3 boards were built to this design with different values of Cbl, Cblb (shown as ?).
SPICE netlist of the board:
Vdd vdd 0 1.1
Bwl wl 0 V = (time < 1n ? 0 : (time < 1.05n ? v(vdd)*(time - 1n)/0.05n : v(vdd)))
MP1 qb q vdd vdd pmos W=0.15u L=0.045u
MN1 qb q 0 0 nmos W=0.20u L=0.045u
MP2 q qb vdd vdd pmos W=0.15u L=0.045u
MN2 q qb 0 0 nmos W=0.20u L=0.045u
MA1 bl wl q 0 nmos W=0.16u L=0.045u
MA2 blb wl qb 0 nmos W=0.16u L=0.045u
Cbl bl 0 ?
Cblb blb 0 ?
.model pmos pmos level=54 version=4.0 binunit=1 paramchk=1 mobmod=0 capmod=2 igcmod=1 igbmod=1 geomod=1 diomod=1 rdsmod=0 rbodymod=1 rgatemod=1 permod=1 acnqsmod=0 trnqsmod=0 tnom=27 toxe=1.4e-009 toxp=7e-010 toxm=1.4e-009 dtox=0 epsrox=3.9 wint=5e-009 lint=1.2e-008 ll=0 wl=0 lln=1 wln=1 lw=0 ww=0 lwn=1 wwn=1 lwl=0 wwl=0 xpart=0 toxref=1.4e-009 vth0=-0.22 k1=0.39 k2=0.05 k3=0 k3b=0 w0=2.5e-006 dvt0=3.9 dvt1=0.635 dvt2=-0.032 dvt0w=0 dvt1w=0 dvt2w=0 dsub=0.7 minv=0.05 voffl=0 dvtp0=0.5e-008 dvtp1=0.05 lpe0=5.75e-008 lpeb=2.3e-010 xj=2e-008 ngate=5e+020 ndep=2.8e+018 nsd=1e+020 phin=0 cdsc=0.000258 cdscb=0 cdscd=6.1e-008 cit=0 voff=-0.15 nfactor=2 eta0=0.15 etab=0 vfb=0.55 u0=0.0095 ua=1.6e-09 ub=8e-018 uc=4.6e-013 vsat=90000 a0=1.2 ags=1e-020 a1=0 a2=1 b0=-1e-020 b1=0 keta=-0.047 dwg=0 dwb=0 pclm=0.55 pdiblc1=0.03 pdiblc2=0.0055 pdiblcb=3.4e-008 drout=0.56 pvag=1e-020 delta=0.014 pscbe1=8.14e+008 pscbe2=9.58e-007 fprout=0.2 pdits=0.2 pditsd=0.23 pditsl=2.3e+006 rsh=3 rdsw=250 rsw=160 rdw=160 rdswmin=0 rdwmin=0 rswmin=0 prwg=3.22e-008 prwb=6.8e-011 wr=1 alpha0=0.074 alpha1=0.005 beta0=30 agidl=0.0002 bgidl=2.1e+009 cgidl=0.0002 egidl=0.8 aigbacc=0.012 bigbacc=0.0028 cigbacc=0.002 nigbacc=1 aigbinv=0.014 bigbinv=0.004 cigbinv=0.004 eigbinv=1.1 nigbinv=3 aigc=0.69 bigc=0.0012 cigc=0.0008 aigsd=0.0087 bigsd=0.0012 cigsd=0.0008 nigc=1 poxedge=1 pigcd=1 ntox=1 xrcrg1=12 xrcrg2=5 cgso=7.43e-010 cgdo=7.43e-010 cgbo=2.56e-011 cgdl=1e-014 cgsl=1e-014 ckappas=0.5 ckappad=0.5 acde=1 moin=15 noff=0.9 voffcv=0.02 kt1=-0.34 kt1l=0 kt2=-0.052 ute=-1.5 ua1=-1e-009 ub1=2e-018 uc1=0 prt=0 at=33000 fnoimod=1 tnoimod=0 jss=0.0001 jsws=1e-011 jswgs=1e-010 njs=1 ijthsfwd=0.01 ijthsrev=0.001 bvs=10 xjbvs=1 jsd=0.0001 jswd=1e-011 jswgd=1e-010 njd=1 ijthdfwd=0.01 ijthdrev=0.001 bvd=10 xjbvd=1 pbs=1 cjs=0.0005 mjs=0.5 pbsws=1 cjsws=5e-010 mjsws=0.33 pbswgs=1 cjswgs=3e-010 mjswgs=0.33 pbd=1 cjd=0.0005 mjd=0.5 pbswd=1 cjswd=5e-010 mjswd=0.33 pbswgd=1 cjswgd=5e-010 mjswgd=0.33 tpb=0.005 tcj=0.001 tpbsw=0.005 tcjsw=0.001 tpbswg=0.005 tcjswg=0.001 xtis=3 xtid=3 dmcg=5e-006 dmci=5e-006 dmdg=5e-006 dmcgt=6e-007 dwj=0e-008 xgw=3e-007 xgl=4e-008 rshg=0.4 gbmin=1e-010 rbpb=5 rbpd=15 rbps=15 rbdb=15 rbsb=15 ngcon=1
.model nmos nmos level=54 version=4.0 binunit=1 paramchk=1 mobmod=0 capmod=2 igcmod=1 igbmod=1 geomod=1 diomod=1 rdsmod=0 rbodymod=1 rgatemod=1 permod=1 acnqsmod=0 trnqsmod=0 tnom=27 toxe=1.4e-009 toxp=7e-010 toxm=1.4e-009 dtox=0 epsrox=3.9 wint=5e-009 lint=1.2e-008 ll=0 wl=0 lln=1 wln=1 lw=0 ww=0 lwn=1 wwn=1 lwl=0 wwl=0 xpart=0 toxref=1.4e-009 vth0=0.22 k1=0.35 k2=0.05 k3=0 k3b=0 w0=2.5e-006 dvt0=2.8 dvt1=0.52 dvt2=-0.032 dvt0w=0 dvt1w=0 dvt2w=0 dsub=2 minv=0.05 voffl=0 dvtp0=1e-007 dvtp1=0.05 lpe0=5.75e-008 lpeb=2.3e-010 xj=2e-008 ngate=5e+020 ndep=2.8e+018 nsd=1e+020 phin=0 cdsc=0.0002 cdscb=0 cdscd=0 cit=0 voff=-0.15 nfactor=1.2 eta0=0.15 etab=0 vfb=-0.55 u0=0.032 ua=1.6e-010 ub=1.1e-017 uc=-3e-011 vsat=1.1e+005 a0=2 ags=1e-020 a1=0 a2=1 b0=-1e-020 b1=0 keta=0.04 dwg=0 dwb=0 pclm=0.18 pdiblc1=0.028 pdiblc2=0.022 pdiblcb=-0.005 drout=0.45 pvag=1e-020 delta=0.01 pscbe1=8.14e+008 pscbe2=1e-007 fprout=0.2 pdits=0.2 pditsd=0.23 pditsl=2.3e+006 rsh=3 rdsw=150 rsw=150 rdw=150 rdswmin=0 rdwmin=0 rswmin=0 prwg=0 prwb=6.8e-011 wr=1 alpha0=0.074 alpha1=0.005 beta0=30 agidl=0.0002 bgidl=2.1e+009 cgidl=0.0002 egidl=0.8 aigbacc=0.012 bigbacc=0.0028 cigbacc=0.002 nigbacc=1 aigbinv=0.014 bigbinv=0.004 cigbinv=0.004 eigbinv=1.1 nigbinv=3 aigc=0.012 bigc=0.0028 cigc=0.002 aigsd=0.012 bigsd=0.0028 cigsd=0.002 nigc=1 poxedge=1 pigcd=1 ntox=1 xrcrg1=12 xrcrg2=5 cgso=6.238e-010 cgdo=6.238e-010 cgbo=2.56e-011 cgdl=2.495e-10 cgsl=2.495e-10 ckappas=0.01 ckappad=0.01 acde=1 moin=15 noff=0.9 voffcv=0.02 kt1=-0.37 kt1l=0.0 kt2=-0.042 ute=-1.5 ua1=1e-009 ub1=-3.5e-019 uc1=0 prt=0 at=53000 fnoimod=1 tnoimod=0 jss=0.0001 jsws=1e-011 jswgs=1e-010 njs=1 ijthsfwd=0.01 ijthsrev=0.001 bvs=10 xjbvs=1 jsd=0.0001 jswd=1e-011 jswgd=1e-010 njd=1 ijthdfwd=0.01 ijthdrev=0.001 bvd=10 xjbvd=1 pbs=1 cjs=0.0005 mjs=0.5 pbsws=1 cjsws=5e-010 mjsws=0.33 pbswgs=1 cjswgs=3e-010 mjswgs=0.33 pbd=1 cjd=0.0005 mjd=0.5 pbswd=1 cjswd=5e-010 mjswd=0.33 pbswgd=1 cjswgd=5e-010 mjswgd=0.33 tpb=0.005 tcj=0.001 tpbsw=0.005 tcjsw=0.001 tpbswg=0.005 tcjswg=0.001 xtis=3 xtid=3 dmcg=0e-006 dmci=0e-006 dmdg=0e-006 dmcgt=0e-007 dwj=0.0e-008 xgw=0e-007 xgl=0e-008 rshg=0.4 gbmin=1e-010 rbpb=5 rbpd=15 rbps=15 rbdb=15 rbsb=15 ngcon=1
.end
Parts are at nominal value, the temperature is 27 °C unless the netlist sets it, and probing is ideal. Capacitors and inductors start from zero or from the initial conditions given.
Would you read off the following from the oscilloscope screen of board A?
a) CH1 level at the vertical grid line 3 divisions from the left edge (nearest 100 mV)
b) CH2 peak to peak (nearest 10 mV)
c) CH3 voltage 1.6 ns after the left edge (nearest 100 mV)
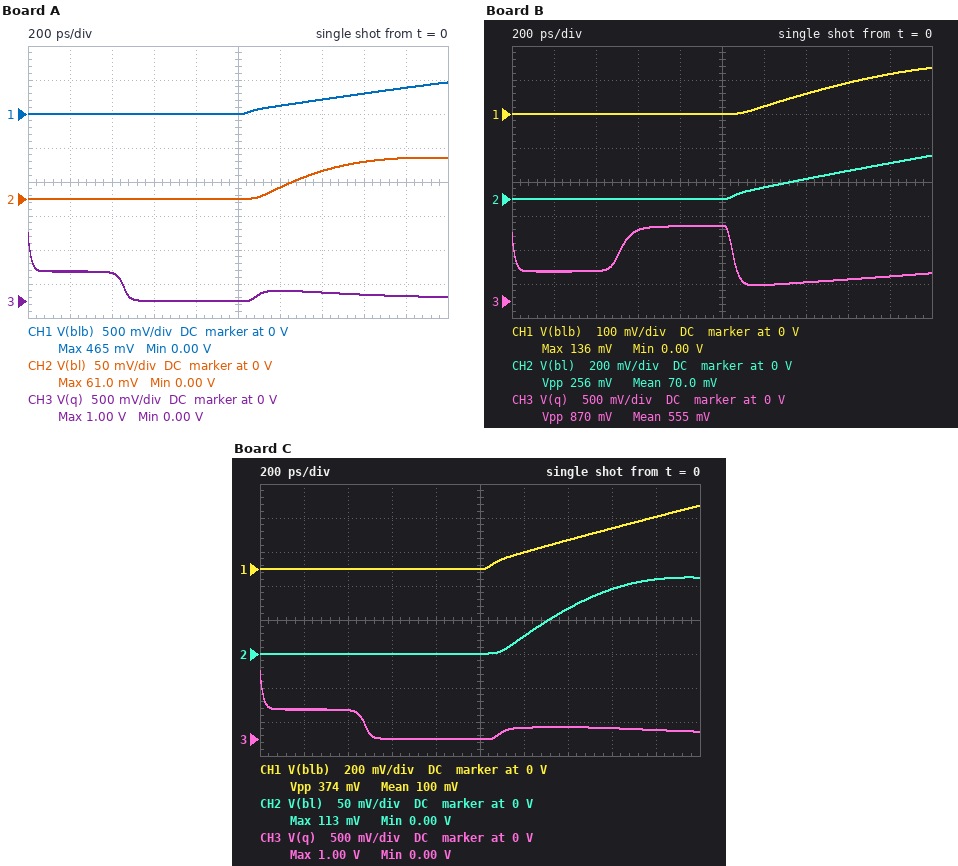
0 V
60 mV
100 mV
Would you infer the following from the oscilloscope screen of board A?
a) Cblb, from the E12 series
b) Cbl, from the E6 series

120 fF
330 fF
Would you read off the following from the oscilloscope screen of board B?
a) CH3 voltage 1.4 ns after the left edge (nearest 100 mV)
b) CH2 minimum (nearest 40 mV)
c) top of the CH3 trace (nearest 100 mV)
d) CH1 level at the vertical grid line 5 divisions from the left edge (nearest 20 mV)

300 mV
0 V
1.1 V
0 V
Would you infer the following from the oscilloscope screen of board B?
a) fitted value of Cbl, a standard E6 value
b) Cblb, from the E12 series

220 fF
270 fF
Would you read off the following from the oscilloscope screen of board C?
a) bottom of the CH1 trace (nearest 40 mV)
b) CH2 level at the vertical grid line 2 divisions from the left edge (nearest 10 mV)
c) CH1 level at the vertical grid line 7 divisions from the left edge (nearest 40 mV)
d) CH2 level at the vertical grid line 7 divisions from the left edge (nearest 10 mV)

0 V
0 V
160 mV
70 mV
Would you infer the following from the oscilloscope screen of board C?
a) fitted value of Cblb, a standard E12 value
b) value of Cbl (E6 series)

150 fF
220 fF
